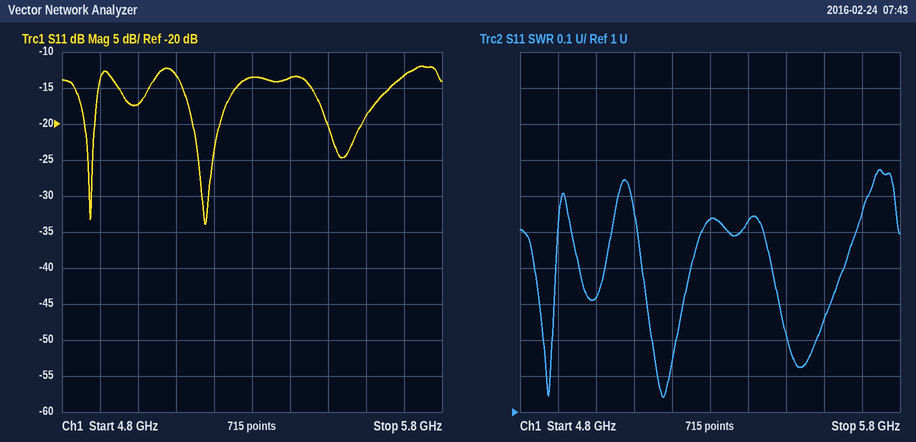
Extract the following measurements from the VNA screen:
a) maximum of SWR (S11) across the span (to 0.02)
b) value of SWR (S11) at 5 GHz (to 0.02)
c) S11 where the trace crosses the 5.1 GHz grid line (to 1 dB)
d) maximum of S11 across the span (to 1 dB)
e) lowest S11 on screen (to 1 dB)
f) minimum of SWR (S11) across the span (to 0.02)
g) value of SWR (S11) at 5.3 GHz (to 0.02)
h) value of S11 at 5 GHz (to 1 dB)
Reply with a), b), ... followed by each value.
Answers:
a) 1.68
b) 1.32
c) -13 dB
d) -12 dB
e) -34 dB
f) 1.04
g) 1.54
h) -17 dB
